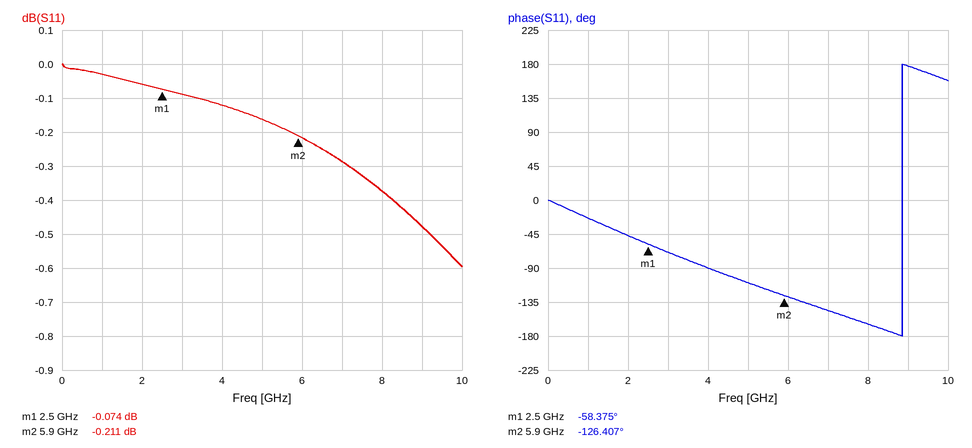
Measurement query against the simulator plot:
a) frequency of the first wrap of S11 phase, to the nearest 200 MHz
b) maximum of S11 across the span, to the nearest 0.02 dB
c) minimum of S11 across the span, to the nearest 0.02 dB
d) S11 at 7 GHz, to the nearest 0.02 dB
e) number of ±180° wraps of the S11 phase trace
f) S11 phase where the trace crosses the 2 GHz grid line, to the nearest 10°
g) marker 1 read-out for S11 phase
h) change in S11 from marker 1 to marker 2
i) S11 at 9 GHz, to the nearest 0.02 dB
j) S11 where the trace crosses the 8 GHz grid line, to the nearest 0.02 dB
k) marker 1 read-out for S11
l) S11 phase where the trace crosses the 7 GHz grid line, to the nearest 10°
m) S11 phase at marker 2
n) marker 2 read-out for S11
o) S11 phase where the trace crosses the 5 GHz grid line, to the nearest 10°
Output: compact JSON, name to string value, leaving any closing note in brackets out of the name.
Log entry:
{"frequency of the first wrap of S11 phase, to the nearest 200 MHz": "8.8 GHz", "maximum of S11 across the span, to the nearest 0.02 dB": "0.00 dB", "minimum of S11 across the span, to the nearest 0.02 dB": "-0.60 dB", "S11 at 7 GHz, to the nearest 0.02 dB": "-0.28 dB", "number of ±180° wraps of the S11 phase trace": "1", "S11 phase where the trace crosses the 2 GHz grid line, to the nearest 10°": "-50°", "marker 1 read-out for S11 phase": "-58.375°", "change in S11 from marker 1 to marker 2": "-0.137 dB", "S11 at 9 GHz, to the nearest 0.02 dB": "-0.48 dB", "S11 where the trace crosses the 8 GHz grid line, to the nearest 0.02 dB": "-0.38 dB", "marker 1 read-out for S11": "-0.074 dB", "S11 phase where the trace crosses the 7 GHz grid line, to the nearest 10°": "-150°", "S11 phase at marker 2": "-126.407°", "marker 2 read-out for S11": "-0.211 dB", "S11 phase where the trace crosses the 5 GHz grid line, to the nearest 10°": "-110°"}
